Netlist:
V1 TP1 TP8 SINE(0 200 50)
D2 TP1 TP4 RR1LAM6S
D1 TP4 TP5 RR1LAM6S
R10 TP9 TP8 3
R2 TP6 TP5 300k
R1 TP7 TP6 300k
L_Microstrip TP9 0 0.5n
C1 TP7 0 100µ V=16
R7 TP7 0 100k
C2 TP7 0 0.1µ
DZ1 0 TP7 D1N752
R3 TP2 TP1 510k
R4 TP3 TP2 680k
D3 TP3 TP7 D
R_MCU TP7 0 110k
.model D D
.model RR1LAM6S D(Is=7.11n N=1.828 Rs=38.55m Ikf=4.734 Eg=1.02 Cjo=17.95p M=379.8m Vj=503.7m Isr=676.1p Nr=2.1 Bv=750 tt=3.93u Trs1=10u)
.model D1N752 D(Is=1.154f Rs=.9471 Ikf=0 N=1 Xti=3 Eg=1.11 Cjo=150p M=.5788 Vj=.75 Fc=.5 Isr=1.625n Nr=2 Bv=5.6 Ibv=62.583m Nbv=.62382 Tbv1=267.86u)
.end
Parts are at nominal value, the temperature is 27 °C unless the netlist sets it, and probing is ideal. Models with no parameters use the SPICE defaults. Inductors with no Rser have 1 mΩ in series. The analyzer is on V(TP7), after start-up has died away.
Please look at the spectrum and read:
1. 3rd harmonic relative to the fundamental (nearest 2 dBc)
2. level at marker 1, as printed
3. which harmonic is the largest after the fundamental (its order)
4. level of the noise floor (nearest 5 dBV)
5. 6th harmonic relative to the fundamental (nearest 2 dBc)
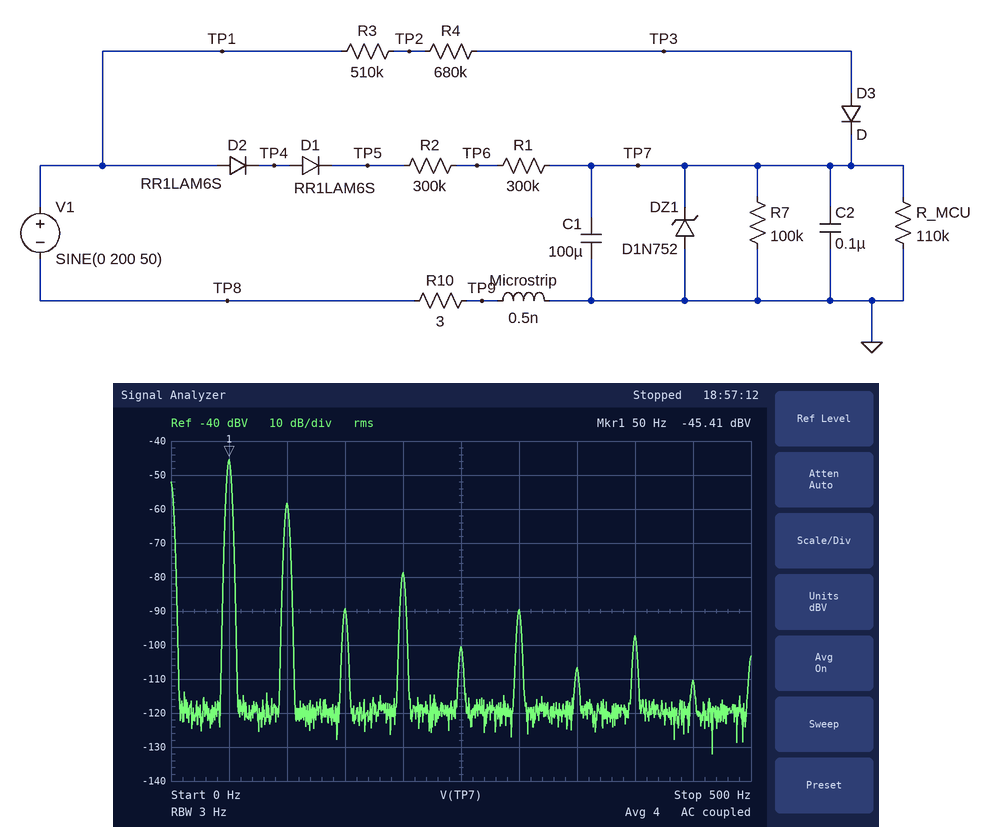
-44 dBc
-45.41 dBV
2
-120 dBV
-44 dBc
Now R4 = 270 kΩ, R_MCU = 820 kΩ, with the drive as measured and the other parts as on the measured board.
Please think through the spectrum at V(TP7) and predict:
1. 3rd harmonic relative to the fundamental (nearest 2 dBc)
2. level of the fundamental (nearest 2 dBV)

-40 dBc
-44 dBV
